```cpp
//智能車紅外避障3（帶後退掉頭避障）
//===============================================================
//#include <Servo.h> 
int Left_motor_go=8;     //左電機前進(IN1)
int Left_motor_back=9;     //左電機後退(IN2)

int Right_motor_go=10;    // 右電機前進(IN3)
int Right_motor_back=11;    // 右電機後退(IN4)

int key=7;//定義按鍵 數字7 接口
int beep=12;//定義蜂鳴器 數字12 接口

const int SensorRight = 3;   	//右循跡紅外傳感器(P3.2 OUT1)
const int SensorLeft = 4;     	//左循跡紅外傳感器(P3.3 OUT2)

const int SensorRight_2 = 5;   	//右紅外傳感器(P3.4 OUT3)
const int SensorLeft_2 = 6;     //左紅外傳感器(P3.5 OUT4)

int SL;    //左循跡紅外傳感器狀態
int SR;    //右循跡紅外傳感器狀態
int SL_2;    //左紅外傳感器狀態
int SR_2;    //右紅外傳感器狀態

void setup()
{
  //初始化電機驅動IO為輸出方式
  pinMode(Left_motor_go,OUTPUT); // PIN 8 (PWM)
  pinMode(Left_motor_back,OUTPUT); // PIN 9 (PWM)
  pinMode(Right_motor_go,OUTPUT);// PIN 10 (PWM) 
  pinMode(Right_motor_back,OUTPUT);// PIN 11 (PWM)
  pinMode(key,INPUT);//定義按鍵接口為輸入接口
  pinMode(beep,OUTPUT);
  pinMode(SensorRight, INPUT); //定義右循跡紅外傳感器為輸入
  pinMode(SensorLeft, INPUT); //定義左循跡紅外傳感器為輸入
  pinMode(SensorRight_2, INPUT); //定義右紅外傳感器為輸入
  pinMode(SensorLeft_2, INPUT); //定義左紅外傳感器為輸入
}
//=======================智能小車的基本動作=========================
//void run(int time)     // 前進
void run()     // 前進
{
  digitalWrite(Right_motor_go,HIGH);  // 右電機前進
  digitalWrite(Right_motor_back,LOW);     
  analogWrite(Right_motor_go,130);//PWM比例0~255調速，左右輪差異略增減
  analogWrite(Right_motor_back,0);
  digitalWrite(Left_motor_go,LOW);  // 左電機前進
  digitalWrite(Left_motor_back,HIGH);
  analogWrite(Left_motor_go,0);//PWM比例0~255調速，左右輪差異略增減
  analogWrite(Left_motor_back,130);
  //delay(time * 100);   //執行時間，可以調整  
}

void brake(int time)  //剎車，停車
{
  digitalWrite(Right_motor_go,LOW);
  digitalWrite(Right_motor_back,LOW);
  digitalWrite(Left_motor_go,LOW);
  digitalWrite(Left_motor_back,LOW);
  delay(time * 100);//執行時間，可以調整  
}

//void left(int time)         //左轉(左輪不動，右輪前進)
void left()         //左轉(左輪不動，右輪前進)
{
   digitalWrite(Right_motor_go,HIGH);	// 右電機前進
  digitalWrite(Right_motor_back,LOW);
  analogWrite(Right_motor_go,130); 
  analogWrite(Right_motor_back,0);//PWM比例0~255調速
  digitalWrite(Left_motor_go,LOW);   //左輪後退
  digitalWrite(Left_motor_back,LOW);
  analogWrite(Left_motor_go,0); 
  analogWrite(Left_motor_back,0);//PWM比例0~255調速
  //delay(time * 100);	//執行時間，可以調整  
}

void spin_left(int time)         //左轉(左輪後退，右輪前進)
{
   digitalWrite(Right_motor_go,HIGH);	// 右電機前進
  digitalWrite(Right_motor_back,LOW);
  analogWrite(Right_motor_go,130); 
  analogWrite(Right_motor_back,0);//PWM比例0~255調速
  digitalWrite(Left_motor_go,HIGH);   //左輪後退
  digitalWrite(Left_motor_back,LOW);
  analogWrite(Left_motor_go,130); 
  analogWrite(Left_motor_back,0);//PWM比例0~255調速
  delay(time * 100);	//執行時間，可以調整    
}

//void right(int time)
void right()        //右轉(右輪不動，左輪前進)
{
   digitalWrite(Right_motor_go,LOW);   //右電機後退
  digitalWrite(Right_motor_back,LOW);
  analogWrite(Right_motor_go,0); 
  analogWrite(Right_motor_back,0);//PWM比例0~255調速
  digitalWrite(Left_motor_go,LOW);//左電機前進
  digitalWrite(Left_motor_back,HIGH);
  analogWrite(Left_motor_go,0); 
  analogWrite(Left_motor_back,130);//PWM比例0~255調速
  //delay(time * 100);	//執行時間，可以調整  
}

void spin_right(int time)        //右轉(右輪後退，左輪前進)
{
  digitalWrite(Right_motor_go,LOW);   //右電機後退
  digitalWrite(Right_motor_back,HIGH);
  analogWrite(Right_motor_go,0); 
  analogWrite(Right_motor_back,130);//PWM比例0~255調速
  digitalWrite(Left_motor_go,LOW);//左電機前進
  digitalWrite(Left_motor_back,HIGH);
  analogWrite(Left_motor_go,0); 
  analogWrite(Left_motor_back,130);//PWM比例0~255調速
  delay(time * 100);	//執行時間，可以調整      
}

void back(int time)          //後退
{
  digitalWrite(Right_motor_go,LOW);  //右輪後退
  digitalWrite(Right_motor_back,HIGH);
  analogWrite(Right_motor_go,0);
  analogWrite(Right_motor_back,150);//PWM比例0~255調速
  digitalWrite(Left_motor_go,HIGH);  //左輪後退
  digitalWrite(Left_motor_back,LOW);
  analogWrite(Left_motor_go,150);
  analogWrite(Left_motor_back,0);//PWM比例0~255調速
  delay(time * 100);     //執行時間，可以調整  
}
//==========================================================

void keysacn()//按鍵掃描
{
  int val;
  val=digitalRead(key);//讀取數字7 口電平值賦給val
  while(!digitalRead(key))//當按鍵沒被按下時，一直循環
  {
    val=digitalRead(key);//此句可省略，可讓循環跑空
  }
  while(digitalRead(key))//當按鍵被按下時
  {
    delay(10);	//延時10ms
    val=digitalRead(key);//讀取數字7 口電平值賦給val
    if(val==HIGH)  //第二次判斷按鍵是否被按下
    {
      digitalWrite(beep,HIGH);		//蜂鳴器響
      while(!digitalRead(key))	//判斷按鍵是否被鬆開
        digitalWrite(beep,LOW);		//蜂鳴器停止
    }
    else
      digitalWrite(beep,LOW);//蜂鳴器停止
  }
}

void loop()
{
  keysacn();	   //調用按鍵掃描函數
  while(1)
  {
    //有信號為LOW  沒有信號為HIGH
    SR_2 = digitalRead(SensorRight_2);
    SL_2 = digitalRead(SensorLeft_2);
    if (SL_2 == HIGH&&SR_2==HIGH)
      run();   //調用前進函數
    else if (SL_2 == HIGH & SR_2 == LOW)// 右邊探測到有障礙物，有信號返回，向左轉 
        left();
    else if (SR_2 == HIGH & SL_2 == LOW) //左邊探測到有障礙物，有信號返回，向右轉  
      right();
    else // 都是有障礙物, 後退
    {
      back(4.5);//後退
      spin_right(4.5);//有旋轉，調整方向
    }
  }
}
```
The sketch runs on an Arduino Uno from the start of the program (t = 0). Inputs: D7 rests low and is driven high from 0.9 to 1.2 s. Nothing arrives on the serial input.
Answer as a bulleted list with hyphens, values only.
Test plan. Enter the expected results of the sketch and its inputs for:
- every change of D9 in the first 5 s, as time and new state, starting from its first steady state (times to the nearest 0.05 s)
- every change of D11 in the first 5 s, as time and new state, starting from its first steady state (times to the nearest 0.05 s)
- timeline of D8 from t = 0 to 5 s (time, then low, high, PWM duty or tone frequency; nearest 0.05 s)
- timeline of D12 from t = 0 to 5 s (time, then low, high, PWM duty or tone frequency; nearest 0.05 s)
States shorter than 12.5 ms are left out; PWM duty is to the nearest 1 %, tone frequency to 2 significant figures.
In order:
- 0 s low; 1.6 s PWM 51 %; 2 s low; 2.4 s PWM 51 %; 2.8 s low; 3.2 s PWM 51 %; 3.6 s low; 4 s PWM 51 %; 4.4 s low; 4.8 s PWM 51 %
- 0 s low; 1.2 s PWM 59 %; 1.6 s PWM 51 %; 2 s PWM 59 %; 2.4 s PWM 51 %; 2.8 s PWM 59 %; 3.2 s PWM 51 %; 3.6 s PWM 59 %; 4 s PWM 51 %; 4.4 s PWM 59 %; 4.8 s PWM 51 %
- 0 s low; 1.2 s high; 1.6 s low; 2 s high; 2.4 s low; 2.8 s high; 3.2 s low; 3.6 s high; 4 s low; 4.4 s high; 4.8 s low
- 0 s low; 0.9 s high; 1.2 s low
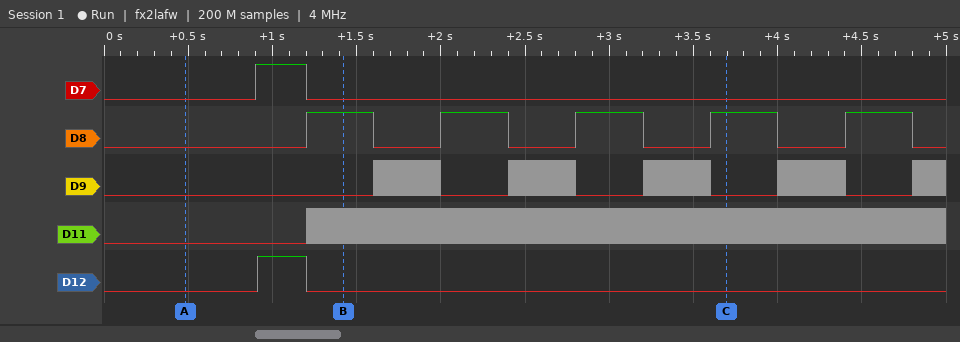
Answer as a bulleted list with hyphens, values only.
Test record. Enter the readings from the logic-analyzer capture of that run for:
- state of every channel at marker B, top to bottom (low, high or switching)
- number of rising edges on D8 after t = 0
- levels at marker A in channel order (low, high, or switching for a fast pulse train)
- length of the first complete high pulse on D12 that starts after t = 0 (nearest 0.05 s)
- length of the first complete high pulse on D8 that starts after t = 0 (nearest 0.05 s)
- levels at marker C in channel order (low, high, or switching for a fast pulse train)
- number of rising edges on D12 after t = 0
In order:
- D7 low, D8 high, D9 low, D11 switching, D12 low
- 5
- D7 low, D8 low, D9 low, D11 low, D12 low
- 0.30 s
- 0.40 s
- D7 low, D8 high, D9 low, D11 switching, D12 low
- 1
